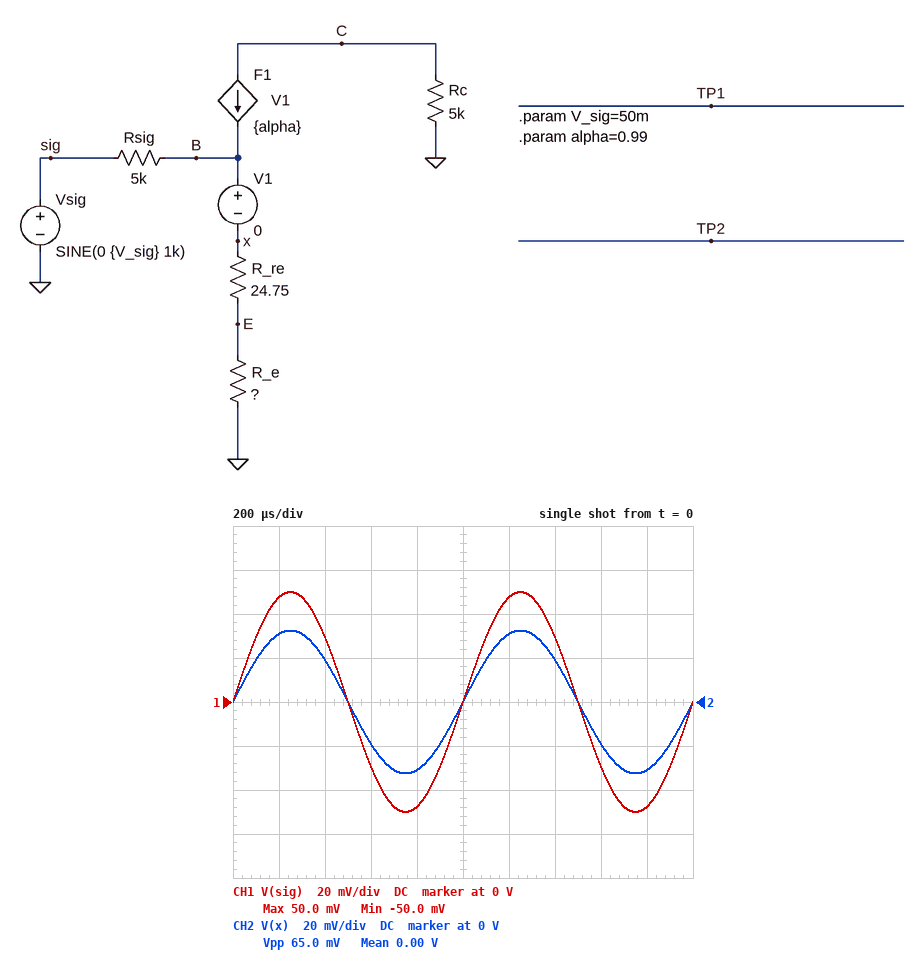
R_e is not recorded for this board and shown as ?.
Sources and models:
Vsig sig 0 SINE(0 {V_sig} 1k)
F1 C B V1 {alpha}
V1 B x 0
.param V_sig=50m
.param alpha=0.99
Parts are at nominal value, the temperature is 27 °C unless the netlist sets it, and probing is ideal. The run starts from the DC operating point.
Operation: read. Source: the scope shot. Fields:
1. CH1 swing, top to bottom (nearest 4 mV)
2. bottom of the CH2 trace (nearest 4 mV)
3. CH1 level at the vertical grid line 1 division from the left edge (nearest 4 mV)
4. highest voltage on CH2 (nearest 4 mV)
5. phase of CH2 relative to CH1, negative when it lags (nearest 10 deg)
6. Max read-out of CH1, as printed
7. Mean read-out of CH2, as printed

100 mV
-32 mV
48 mV
32 mV
0 deg
50.0 mV
0.00 V
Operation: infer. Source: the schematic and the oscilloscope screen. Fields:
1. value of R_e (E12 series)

68 Ω
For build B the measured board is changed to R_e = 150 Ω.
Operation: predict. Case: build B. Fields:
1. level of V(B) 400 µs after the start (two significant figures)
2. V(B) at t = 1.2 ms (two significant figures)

23 mV
37 mV
